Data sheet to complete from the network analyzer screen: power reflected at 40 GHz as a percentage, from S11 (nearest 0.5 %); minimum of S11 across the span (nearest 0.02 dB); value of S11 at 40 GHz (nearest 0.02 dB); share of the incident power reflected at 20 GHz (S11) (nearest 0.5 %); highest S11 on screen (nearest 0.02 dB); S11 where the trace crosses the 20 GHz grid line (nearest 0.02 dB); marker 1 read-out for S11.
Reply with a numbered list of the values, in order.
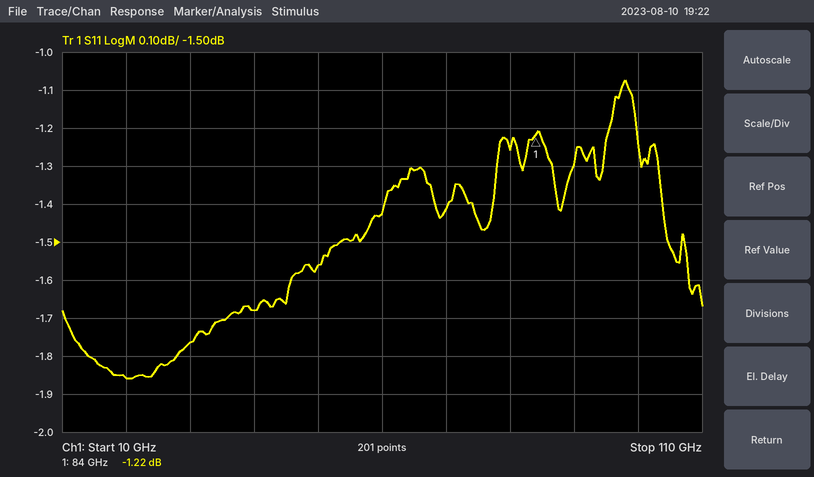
1. 68.0 %
2. -1.86 dB
3. -1.68 dB
4. 65.0 %
5. -1.08 dB
6. -1.86 dB
7. -1.22 dB
